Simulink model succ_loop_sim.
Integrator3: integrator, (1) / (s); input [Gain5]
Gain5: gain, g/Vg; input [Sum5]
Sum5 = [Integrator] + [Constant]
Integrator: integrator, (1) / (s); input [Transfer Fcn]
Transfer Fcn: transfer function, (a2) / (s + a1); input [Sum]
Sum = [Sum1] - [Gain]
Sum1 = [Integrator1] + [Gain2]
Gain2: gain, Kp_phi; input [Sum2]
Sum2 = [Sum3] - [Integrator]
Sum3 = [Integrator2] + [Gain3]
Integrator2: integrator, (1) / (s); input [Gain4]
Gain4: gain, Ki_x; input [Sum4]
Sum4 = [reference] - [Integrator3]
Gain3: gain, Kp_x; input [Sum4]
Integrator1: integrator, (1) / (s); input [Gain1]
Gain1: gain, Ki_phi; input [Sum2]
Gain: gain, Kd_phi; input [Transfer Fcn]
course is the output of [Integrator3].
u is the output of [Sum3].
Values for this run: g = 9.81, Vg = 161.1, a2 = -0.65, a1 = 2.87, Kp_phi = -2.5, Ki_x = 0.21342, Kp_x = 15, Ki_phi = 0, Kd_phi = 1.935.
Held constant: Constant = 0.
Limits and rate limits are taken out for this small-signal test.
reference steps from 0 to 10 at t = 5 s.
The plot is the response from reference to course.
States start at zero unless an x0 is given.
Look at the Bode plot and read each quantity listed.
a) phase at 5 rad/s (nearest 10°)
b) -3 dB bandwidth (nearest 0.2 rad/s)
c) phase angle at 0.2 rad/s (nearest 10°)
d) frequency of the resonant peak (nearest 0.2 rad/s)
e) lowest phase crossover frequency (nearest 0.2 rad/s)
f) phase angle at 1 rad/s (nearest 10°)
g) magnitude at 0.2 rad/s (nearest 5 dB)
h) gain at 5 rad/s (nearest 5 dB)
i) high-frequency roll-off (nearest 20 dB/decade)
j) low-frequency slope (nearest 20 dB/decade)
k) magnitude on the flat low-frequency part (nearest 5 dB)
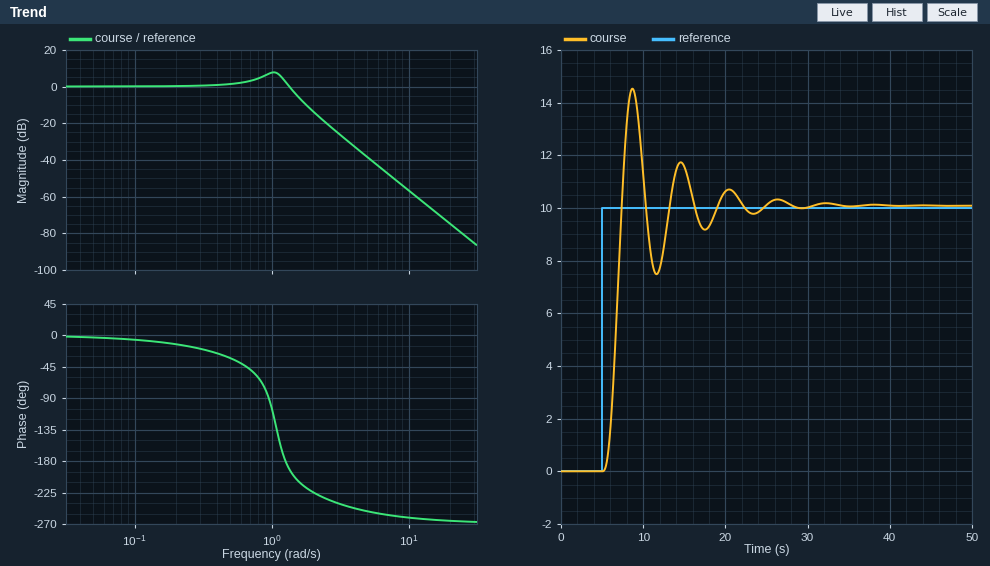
-250°
1.4 rad/s
-10°
1.0 rad/s
1.2 rad/s
-100°
0 dB
-40 dB
-60 dB/decade
0 dB/decade
0 dB
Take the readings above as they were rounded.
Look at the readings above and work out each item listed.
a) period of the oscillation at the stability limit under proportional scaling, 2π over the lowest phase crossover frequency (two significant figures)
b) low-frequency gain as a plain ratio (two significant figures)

5.2 s
1.0
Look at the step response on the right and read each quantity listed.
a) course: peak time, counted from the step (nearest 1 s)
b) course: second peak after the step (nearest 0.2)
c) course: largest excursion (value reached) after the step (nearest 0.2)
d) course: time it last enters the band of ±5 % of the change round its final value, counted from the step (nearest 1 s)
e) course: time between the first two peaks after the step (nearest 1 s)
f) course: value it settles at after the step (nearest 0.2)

4 s
11.8
14.6
16 s
6 s
10.0
